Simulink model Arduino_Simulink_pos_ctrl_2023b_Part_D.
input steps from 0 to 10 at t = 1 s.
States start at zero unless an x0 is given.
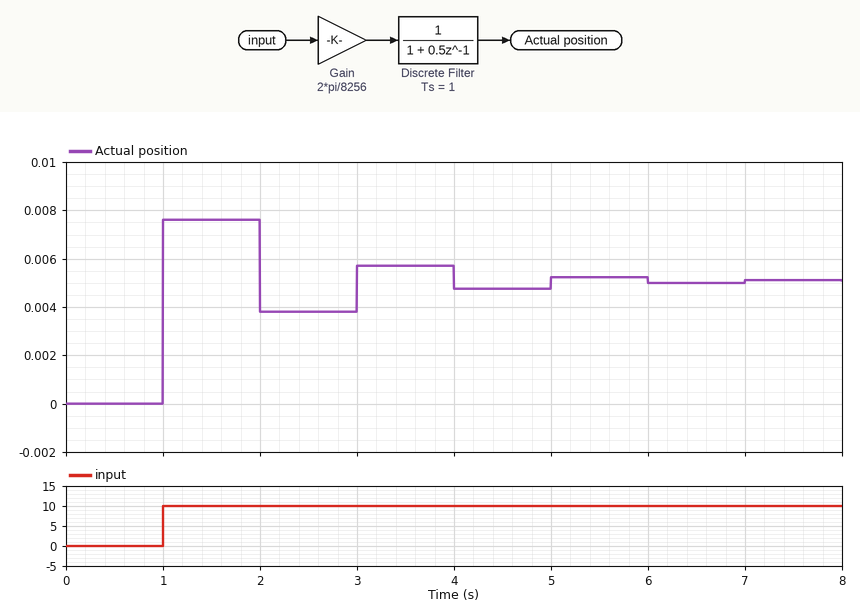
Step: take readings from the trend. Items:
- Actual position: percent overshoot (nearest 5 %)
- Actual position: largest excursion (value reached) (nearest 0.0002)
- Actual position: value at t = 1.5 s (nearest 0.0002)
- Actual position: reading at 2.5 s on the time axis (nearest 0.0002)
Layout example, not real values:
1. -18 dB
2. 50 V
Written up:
1. 50 %
2. 0.0076
3. 0.0076
4. 0.0038
